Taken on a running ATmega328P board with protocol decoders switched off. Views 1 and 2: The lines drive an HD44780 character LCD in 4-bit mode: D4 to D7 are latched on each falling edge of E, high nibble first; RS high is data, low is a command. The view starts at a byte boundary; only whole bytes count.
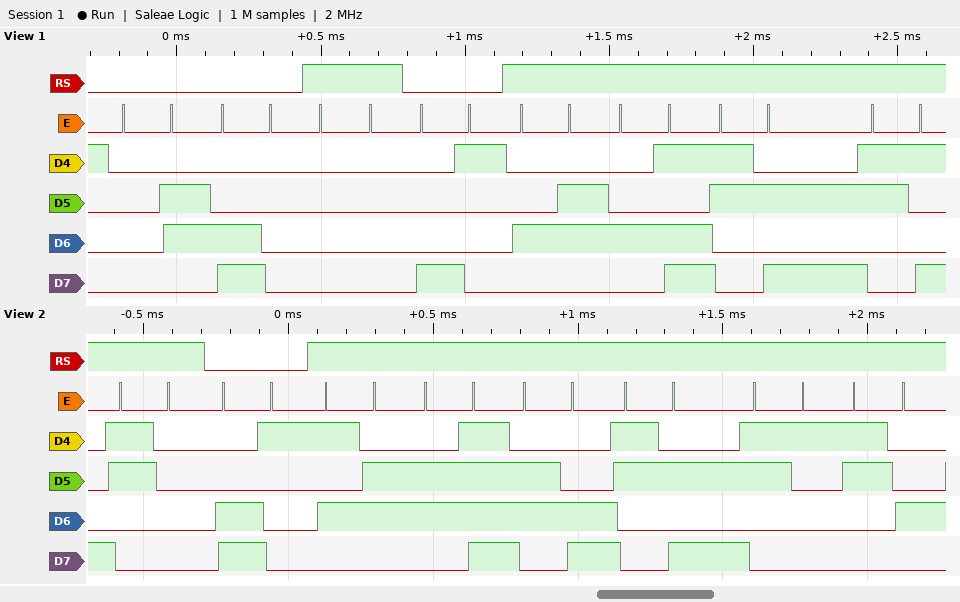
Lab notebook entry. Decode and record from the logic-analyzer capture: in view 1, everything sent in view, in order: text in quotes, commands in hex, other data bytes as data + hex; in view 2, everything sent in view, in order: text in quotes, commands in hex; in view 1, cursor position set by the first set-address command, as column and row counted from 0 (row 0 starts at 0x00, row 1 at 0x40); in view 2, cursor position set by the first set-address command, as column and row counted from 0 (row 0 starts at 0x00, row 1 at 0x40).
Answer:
0x06 0xC0 data 00 0x81 "FM:9"
"0" 0xC1 "Vol:14"
column 0, row 1
column 1, row 1
